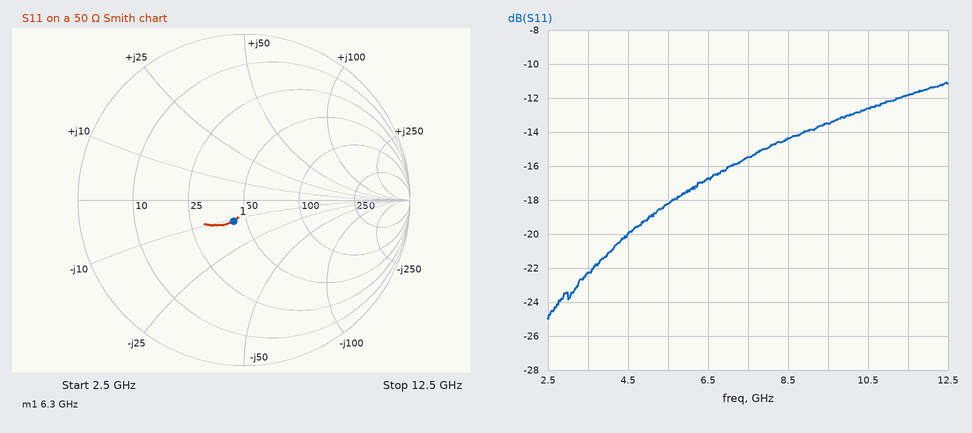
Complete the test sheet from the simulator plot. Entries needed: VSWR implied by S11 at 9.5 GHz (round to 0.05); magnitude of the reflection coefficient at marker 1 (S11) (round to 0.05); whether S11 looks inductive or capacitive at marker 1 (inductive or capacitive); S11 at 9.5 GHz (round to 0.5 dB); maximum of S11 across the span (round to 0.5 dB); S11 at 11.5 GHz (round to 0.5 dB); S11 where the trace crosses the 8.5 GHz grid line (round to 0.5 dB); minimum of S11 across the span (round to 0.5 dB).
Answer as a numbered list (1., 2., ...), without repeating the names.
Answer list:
1. 1.55
2. 0.15
3. capacitive
4. -13.5 dB
5. -11.0 dB
6. -12.0 dB
7. -14.5 dB
8. -25.0 dB
